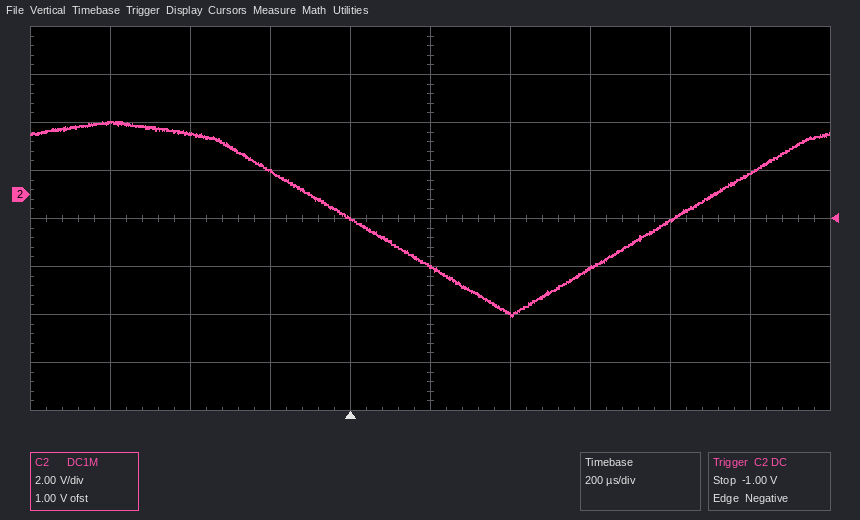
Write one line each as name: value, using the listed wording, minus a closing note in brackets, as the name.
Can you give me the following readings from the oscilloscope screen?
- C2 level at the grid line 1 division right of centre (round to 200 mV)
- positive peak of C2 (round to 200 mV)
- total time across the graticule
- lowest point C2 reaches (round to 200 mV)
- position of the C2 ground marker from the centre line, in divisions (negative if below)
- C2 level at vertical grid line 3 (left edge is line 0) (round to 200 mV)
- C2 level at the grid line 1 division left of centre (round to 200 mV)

C2 level at the grid line 1 division right of centre: -5.0 V
positive peak of C2: 3.0 V
total time across the graticule: 2 ms
lowest point C2 reaches: -5.0 V
position of the C2 ground marker from the centre line, in divisions: +0.5 div
C2 level at vertical grid line 3 (left edge is line 0): 1.0 V
C2 level at the grid line 1 division left of centre: -1.0 V
